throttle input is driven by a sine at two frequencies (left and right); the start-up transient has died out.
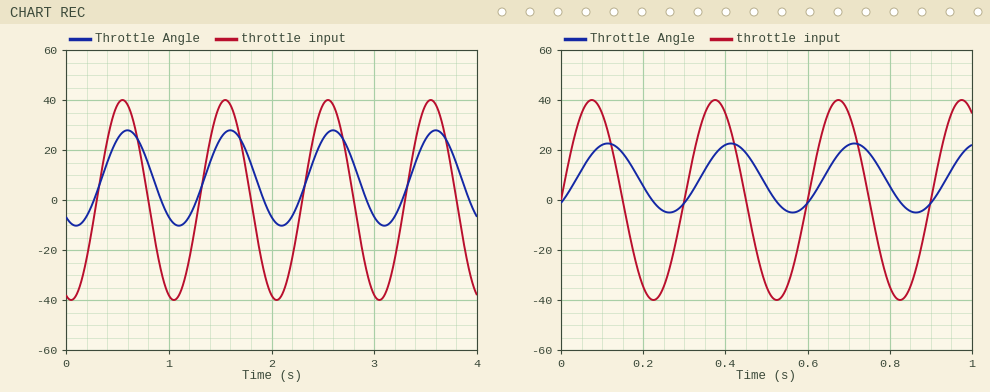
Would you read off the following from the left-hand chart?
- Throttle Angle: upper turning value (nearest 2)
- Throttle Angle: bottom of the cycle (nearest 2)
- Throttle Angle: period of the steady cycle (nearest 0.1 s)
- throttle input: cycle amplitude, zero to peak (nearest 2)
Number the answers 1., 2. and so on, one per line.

1. 28
2. -10
3. 1.0 s
4. 40
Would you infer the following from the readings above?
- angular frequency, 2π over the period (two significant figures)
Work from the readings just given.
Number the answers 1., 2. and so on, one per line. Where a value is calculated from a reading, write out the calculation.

1. 2π / 1 = 6.3 rad/s
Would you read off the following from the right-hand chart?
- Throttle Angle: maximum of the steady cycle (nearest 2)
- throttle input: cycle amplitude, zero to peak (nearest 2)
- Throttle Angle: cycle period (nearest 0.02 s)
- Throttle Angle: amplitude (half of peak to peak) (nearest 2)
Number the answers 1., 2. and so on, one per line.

1. 22
2. 40
3. 0.30 s
4. 14
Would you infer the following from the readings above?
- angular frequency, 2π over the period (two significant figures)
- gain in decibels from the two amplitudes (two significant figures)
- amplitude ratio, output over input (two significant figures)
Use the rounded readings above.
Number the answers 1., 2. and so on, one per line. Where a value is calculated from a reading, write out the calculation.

1. 2π / 0.3 = 21 rad/s
2. 20 log10(14 / 40) = -9.1 dB
3. 14 / 40 = 0.35
